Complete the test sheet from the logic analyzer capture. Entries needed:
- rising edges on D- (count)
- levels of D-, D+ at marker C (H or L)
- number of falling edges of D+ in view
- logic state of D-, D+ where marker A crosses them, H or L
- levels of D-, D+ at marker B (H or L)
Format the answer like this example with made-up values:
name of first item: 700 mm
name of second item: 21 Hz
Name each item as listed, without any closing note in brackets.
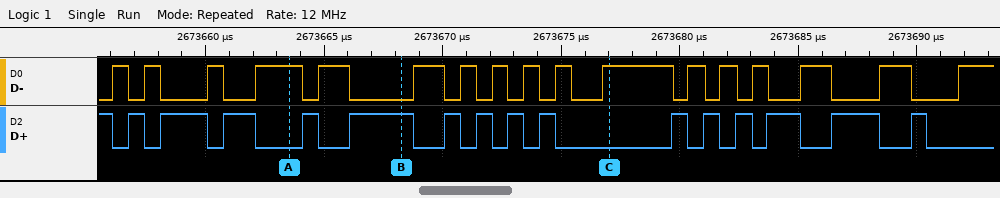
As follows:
rising edges on D-: 17
levels of D-, D+ at marker C: D-=H, D+=L
number of falling edges of D+ in view: 16
logic state of D-, D+ where marker A crosses them, H or L: D-=H, D+=L
levels of D-, D+ at marker B: D-=L, D+=H
